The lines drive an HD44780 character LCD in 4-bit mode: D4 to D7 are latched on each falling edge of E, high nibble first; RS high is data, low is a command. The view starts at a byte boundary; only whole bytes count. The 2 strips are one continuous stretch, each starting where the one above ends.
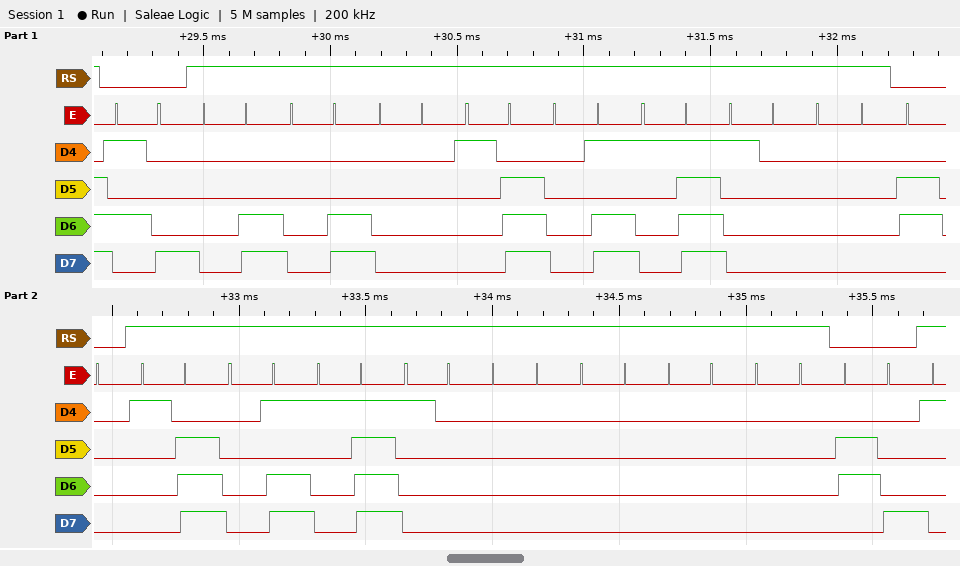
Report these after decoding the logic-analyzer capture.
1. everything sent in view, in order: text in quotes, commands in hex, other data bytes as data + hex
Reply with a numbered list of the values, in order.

1. 0x58 data 0C 0C 00 1E 0D 1F 10 00 0x60 data 1E 0D 1F 10 00 00 00 00 0x68
